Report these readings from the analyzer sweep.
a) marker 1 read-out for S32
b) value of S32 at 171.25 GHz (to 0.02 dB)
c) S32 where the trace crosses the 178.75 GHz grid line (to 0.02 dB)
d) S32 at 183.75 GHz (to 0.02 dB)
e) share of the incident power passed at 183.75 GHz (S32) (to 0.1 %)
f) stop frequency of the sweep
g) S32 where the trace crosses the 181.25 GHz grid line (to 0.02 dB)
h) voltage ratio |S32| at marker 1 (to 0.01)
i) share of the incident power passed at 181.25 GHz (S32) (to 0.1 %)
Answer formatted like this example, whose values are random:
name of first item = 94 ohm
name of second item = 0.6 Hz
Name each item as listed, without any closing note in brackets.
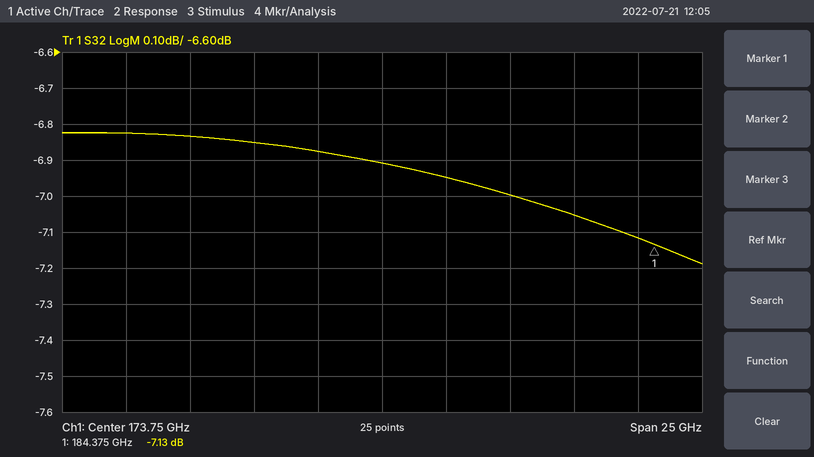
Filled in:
marker 1 read-out for S32 = -7.13 dB
value of S32 at 171.25 GHz = -6.88 dB
S32 where the trace crosses the 178.75 GHz grid line = -7.00 dB
S32 at 183.75 GHz = -7.12 dB
share of the incident power passed at 183.75 GHz (S32) = 19.4 %
stop frequency of the sweep = 186.25 GHz
S32 where the trace crosses the 181.25 GHz grid line = -7.06 dB
voltage ratio |S32| at marker 1 = 0.44
share of the incident power passed at 181.25 GHz (S32) = 19.7 %
